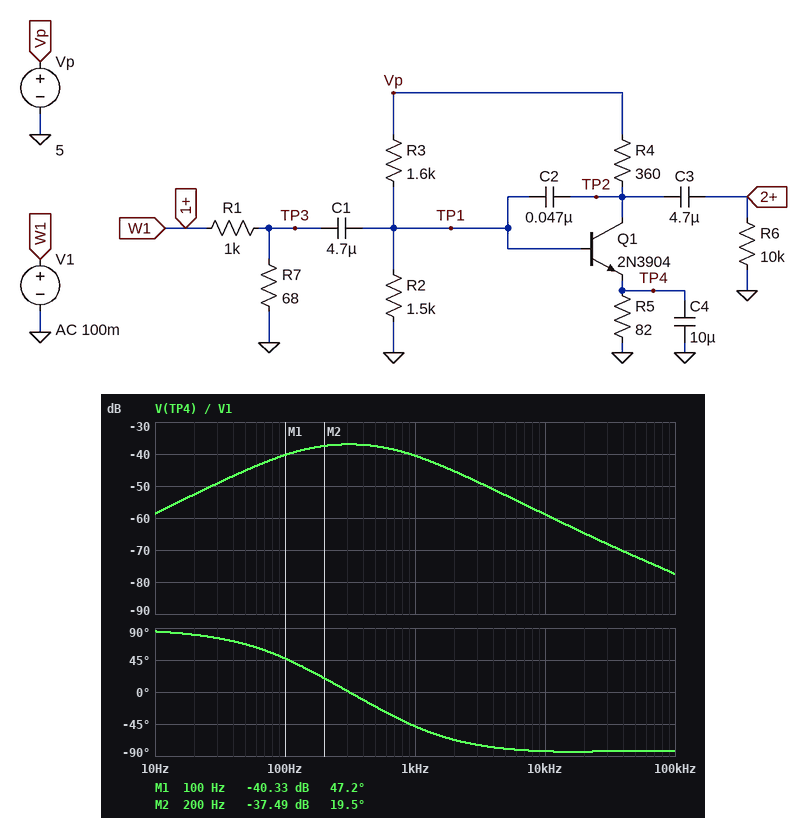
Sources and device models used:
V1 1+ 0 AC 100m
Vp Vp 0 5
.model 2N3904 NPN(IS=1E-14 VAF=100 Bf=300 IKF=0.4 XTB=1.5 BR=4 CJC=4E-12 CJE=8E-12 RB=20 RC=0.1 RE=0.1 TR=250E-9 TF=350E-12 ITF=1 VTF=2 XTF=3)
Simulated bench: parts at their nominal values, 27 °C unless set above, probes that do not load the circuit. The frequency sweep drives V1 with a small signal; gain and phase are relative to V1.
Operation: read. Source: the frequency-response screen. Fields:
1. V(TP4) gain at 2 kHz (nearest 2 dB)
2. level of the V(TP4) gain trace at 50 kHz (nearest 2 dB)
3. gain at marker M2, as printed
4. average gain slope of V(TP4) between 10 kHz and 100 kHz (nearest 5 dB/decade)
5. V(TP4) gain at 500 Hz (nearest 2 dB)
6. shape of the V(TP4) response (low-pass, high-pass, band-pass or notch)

-46 dB
-72 dB
-37.49 dB
-20 dB/decade
-38 dB
band-pass
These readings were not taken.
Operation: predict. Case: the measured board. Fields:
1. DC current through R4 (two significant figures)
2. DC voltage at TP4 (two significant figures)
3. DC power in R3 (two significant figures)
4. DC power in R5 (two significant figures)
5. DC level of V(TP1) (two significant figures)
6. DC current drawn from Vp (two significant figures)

11 mA
980 mV
6.7 mW
12 mW
1.7 V
13 mA
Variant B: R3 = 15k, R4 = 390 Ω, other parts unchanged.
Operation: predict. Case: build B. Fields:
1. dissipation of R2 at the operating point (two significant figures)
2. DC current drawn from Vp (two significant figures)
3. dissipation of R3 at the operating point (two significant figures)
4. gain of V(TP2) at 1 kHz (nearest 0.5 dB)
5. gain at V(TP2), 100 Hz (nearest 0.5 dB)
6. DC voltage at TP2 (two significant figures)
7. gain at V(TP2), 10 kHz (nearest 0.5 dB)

140 µW
300 µA
1.4 mW
-43.5 dB
-62.5 dB
5.0 V
-27.5 dB
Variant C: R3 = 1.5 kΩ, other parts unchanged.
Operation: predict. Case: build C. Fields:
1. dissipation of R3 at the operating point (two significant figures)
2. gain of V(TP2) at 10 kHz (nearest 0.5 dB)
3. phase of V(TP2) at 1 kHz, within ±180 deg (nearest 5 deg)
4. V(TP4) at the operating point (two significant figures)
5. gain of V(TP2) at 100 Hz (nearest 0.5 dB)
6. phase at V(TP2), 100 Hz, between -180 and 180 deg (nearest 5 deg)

7.1 mW
-38.5 dB
-105 deg
990 mV
-43.0 dB
40 deg
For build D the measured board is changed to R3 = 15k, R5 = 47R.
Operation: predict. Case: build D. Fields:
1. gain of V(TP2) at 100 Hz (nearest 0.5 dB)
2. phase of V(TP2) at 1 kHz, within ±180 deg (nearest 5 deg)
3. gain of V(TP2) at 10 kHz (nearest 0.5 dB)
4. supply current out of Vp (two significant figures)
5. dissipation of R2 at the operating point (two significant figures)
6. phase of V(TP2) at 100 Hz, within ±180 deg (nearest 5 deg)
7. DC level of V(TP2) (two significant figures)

-63.0 dB
90 deg
-28.0 dB
300 µA
140 µW
135 deg
5.0 V
